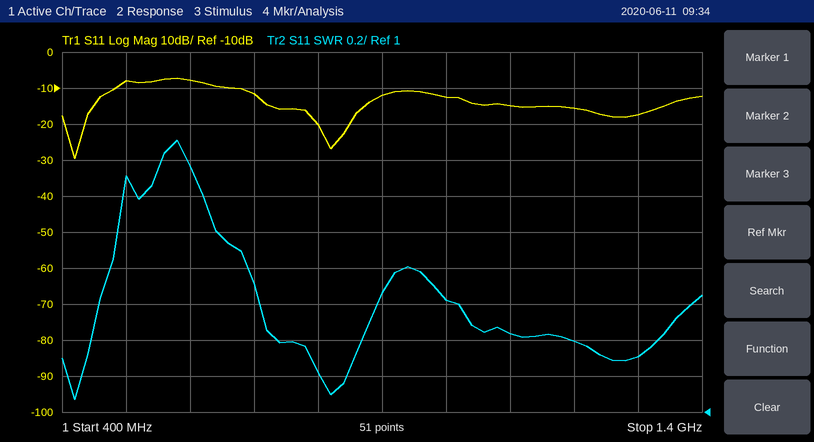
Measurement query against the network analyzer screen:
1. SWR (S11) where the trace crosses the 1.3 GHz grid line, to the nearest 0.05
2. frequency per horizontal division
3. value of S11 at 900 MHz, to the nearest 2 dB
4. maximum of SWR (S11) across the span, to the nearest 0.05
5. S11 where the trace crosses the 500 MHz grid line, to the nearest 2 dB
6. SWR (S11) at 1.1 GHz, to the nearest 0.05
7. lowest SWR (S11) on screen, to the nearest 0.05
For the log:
1.30
100 MHz
-12 dB
2.50
-8 dB
1.45
1.05
